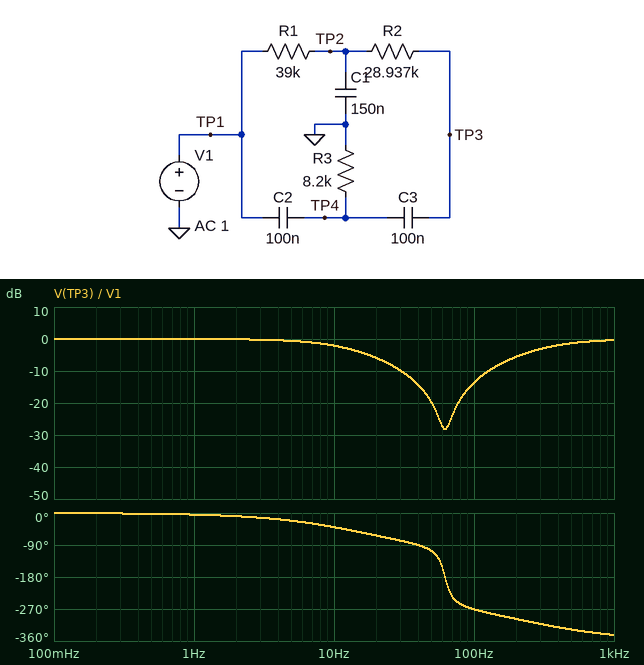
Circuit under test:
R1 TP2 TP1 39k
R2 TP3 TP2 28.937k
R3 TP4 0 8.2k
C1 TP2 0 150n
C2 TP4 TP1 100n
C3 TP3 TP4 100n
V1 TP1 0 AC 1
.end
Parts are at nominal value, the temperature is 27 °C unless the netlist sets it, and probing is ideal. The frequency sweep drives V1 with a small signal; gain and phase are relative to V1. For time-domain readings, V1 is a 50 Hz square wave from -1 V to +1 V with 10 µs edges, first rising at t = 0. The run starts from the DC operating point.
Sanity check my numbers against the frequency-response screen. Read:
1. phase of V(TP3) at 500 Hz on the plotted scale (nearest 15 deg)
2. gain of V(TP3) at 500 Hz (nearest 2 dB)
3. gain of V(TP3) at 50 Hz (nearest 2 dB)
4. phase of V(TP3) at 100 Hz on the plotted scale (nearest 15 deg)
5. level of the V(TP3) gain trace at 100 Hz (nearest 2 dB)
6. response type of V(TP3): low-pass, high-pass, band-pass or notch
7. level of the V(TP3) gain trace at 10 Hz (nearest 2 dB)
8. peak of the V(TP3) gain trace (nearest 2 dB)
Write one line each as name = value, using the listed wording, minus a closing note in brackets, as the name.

phase of V(TP3) at 500 Hz on the plotted scale = -330 deg
gain of V(TP3) at 500 Hz = -2 dB
gain of V(TP3) at 50 Hz = -20 dB
phase of V(TP3) at 100 Hz on the plotted scale = -270 deg
level of the V(TP3) gain trace at 100 Hz = -14 dB
response type of V(TP3): low-pass, high-pass, band-pass or notch = notch
level of the V(TP3) gain trace at 10 Hz = -2 dB
peak of the V(TP3) gain trace = 0 dB
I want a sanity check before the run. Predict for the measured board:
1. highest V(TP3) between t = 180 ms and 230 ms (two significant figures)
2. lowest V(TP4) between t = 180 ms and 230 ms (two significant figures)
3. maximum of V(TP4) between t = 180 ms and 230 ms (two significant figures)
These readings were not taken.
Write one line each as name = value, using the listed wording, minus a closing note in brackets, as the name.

highest V(TP3) between t = 180 ms and 230 ms = 1.7 V
lowest V(TP4) between t = 180 ms and 230 ms = -1.9 V
maximum of V(TP4) between t = 180 ms and 230 ms = 1.9 V
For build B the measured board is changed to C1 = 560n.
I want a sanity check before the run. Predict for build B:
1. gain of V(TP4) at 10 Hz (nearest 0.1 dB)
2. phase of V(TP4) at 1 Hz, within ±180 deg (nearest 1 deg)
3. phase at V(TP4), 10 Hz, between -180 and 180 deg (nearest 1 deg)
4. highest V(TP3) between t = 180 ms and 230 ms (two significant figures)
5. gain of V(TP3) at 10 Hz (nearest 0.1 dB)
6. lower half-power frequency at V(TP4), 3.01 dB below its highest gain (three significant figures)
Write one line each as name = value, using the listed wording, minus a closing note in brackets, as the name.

gain of V(TP4) at 10 Hz = -23.7 dB
phase of V(TP4) at 1 Hz, within ±180 deg = 84 deg
phase at V(TP4), 10 Hz, between -180 and 180 deg = 63 deg
highest V(TP3) between t = 180 ms and 230 ms = 1.9 V
gain of V(TP3) at 10 Hz = -6.1 dB
lower half-power frequency at V(TP4), 3.01 dB below its highest gain = 262 Hz
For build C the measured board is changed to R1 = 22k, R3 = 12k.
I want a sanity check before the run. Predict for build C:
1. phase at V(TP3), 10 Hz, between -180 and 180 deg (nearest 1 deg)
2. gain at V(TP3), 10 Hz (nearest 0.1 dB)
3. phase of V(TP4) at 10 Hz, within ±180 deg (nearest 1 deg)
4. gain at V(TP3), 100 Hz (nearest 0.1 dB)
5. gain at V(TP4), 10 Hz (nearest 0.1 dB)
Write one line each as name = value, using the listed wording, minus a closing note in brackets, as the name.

phase at V(TP3), 10 Hz, between -180 and 180 deg = -28 deg
gain at V(TP3), 10 Hz = -1.2 dB
phase of V(TP4) at 10 Hz, within ±180 deg = 68 deg
gain at V(TP3), 100 Hz = -13.5 dB
gain at V(TP4), 10 Hz = -17.4 dB
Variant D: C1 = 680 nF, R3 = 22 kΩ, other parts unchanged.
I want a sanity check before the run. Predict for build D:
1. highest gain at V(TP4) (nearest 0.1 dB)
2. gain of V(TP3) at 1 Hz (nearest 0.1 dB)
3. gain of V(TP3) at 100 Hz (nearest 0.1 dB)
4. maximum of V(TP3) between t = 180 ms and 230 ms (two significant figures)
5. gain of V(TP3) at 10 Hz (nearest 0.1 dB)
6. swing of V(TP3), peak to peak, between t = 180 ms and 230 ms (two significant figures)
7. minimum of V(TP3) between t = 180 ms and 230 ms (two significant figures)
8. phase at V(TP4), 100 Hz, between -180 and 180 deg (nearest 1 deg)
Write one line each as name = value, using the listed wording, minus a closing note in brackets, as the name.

highest gain at V(TP4) = 0 dB
gain of V(TP3) at 1 Hz = -0.2 dB
gain of V(TP3) at 100 Hz = -6.5 dB
maximum of V(TP3) between t = 180 ms and 230 ms = 1.9 V
gain of V(TP3) at 10 Hz = -7.6 dB
swing of V(TP3), peak to peak, between t = 180 ms and 230 ms = 3.9 V
minimum of V(TP3) between t = 180 ms and 230 ms = -1.9 V
phase at V(TP4), 100 Hz, between -180 and 180 deg = 41 deg
